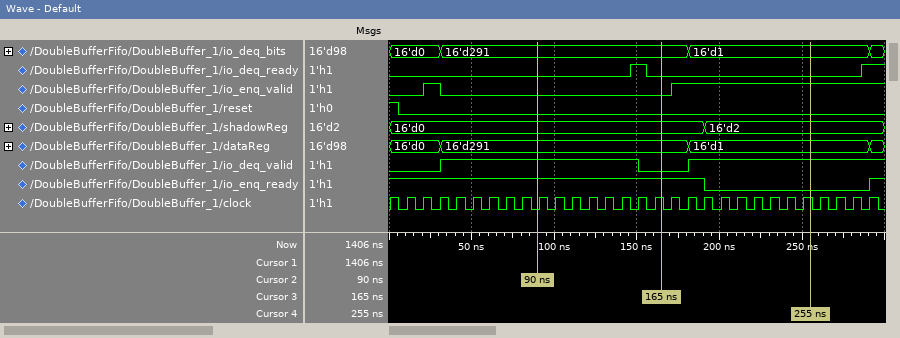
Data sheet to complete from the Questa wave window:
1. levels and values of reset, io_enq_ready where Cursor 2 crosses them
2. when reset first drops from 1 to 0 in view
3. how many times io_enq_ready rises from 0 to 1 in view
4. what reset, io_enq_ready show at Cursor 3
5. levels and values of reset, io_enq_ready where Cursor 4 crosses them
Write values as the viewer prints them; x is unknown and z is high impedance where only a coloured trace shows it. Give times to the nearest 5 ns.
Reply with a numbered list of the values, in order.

1. reset=0, io_enq_ready=1
2. 5 ns
3. 1
4. reset=0, io_enq_ready=1
5. reset=0, io_enq_ready=0
